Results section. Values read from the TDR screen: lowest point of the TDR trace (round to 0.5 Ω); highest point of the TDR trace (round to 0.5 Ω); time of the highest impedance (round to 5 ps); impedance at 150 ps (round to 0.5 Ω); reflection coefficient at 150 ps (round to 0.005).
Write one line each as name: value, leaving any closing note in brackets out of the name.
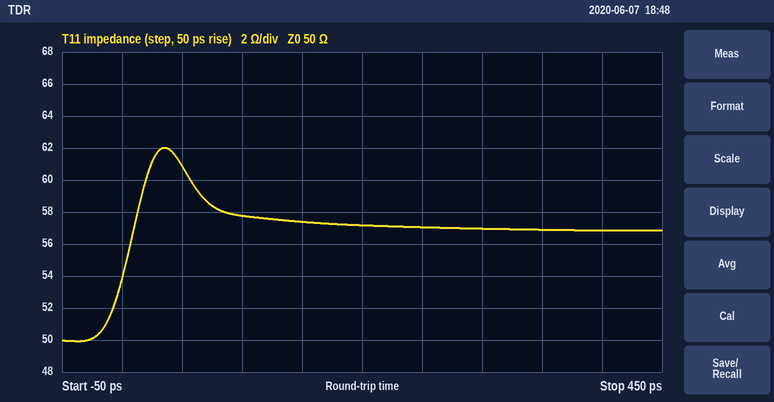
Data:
lowest point of the TDR trace: 50.0 Ω
highest point of the TDR trace: 62.0 Ω
time of the highest impedance: 35 ps
impedance at 150 ps: 57.5 Ω
reflection coefficient at 150 ps: +0.070
